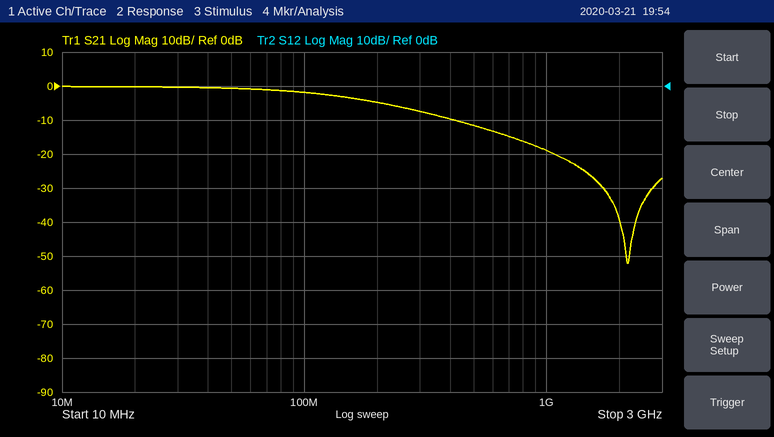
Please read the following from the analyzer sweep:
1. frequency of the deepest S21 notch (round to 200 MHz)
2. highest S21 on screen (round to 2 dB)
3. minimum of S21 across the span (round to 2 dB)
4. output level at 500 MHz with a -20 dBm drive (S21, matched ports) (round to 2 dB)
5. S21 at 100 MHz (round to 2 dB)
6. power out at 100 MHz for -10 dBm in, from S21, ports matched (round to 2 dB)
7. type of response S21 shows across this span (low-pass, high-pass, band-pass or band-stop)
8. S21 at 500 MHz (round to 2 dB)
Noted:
2.2 GHz
0 dB
-52 dB
-32 dBm
-2 dB
-12 dBm
low-pass
-12 dB
